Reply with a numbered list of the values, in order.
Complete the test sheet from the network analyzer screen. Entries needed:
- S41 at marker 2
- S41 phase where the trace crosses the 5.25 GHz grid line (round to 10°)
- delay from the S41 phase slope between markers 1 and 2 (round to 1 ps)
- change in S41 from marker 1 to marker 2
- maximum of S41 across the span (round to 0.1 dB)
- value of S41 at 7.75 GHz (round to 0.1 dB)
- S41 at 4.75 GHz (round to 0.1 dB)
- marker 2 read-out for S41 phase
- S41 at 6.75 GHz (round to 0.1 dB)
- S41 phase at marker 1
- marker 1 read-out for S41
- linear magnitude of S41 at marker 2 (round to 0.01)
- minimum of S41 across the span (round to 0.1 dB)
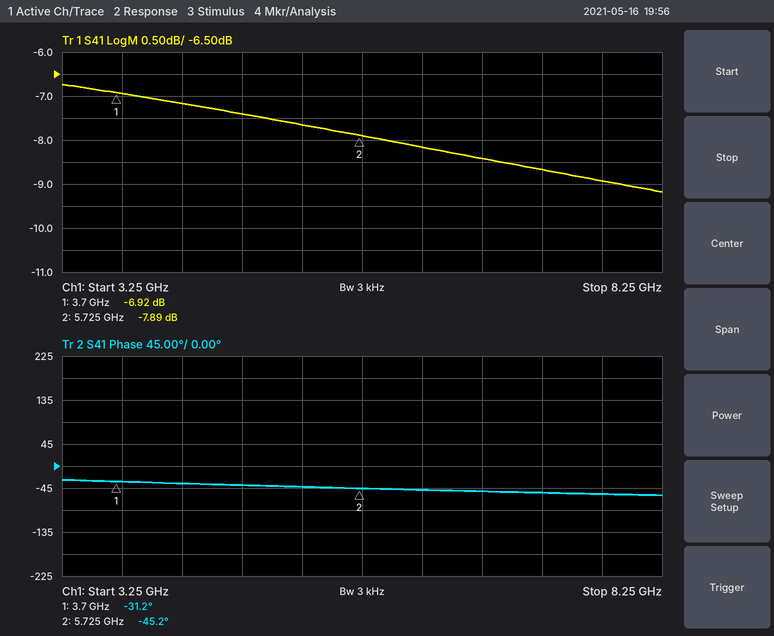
1. -7.89 dB
2. -40°
3. 19 ps
4. -0.97 dB
5. -6.7 dB
6. -8.9 dB
7. -7.4 dB
8. -45.2°
9. -8.4 dB
10. -31.2°
11. -6.92 dB
12. 0.40
13. -9.2 dB
